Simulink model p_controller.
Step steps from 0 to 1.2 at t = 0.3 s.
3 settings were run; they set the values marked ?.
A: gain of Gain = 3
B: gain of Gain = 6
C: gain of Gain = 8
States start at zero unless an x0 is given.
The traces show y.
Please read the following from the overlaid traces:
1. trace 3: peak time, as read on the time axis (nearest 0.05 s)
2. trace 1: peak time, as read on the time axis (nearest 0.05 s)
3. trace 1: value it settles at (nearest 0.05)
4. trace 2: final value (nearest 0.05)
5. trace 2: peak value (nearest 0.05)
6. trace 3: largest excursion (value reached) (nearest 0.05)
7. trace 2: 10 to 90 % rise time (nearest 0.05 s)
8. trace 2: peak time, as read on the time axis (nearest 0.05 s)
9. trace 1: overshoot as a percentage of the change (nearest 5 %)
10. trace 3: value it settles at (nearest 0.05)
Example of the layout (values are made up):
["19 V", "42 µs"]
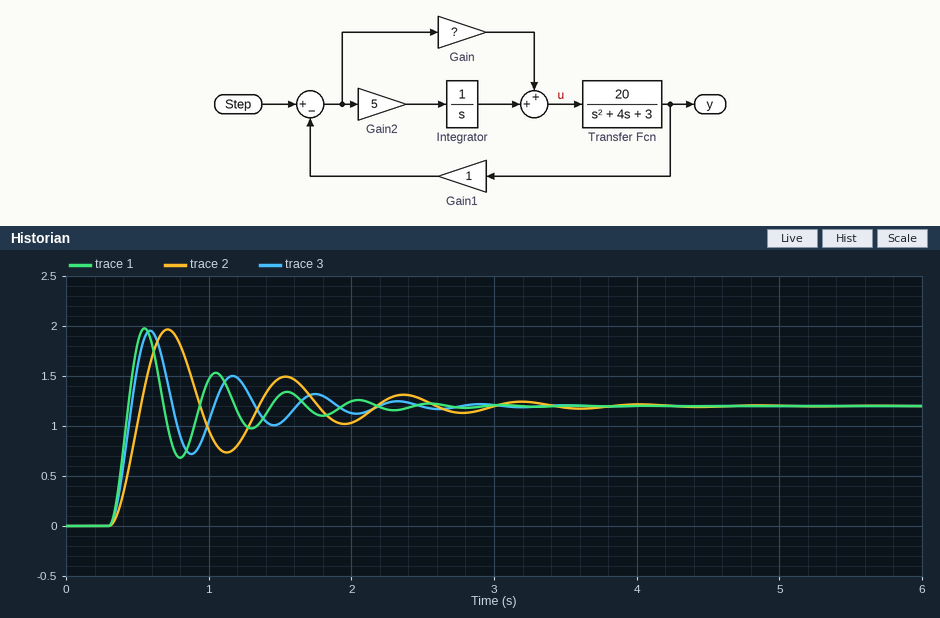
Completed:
["0.60 s", "0.55 s", "1.20", "1.20", "1.95", "1.95", "0.15 s", "0.70 s", "65 %", "1.20"]
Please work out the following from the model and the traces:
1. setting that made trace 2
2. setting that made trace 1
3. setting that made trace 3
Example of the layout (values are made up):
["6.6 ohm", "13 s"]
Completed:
["A", "C", "B"]
